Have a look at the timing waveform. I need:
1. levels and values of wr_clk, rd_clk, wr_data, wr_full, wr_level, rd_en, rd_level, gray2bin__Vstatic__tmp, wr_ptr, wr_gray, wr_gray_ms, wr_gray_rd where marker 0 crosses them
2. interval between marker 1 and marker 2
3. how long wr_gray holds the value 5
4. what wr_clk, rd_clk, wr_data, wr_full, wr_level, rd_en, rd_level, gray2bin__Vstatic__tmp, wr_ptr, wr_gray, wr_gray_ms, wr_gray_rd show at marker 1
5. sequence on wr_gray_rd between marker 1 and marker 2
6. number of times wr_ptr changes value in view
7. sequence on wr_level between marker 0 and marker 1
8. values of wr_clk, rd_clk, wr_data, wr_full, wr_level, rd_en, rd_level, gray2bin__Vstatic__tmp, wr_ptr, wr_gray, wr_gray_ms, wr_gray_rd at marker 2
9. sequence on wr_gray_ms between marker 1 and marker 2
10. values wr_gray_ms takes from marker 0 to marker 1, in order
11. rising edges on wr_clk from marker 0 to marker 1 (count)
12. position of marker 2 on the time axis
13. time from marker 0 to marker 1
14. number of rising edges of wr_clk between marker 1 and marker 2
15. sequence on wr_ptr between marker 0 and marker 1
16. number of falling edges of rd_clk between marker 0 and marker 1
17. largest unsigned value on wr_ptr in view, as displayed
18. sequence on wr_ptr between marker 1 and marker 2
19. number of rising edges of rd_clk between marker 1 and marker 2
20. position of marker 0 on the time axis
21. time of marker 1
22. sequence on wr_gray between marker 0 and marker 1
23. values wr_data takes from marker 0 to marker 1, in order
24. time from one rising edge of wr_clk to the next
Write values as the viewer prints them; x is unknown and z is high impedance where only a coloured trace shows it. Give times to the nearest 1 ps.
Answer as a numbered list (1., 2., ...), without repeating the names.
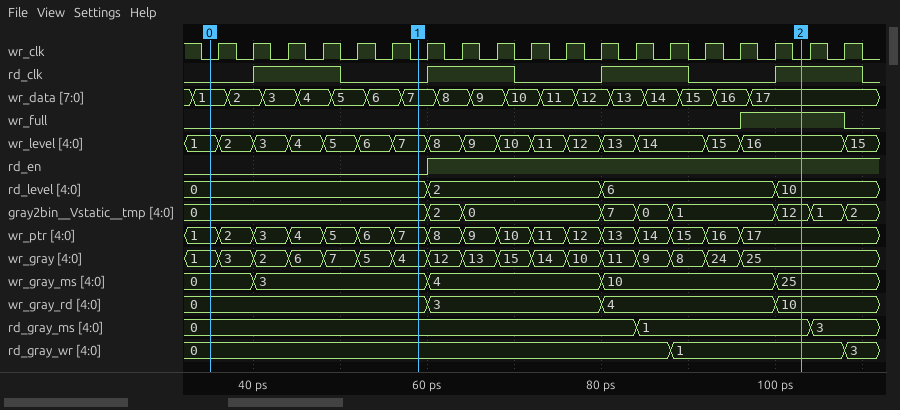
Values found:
1. wr_clk=0, rd_clk=0, wr_data=1, wr_full=0, wr_level=1, rd_en=0, rd_level=0, gray2bin__Vstatic__tmp=0, wr_ptr=1, wr_gray=1, wr_gray_ms=0, wr_gray_rd=0
2. 44 ps
3. 4 ps
4. wr_clk=0, rd_clk=0, wr_data=7, wr_full=0, wr_level=7, rd_en=0, rd_level=0, gray2bin__Vstatic__tmp=0, wr_ptr=7, wr_gray=4, wr_gray_ms=3, wr_gray_rd=0
5. 0, 3, 4, 10
6. 16
7. 1, 2, 3, 4, 5, 6, 7
8. wr_clk=0, rd_clk=1, wr_data=17, wr_full=1, wr_level=16, rd_en=1, rd_level=10, gray2bin__Vstatic__tmp=12, wr_ptr=17, wr_gray=25, wr_gray_ms=25, wr_gray_rd=10
9. 3, 4, 10, 25
10. 0, 3
11. 6
12. 103 ps
13. 24 ps
14. 11
15. 1, 2, 3, 4, 5, 6, 7
16. 1
17. 17
18. 7, 8, 9, 10, 11, 12, 13, 14, 15, 16, 17
19. 3
20. 35 ps
21. 59 ps
22. 1, 3, 2, 6, 7, 5, 4
23. 1, 2, 3, 4, 5, 6, 7
24. 4 ps
